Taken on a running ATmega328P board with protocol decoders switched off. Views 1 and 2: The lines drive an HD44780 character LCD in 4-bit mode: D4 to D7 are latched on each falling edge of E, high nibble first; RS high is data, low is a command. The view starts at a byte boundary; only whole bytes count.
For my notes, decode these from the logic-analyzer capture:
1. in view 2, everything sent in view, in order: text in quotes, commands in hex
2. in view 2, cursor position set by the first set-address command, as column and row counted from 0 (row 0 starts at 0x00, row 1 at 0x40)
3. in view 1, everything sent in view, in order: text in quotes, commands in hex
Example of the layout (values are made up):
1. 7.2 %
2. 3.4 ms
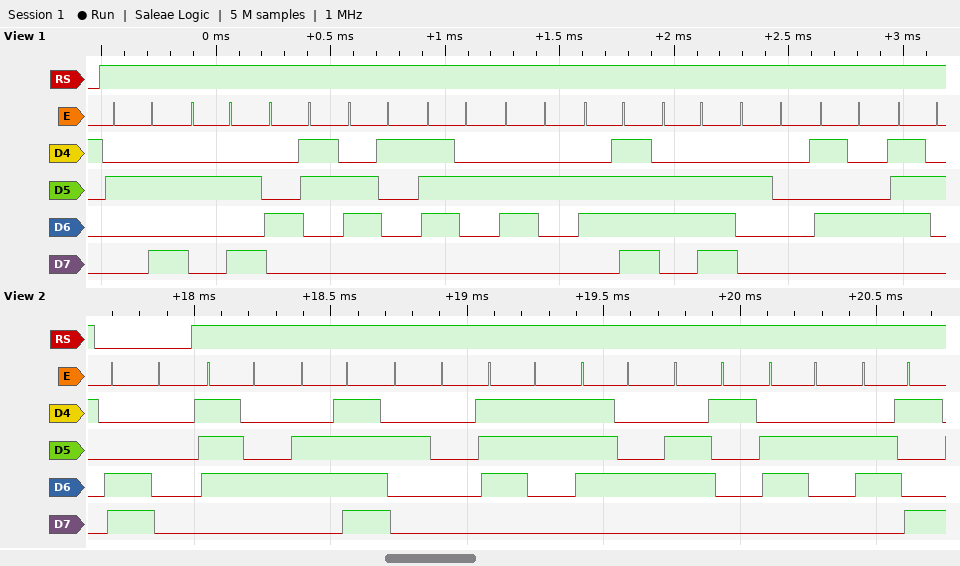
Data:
1. 0xC0 "to stabi"
2. column 0, row 1
3. "**Carbon Tr"
